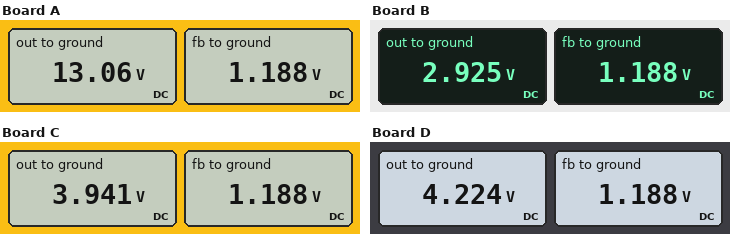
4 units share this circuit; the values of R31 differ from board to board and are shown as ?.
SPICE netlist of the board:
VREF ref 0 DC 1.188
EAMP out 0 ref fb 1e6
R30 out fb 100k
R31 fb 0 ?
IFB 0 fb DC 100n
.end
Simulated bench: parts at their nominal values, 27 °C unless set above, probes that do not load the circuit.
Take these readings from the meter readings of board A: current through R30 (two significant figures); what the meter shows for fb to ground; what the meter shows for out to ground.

120 µA
1.188 V
13.06 V
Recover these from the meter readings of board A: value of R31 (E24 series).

10 kΩ
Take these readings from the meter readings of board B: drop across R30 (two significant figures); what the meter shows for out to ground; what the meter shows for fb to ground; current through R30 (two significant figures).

1.7 V
2.925 V
1.188 V
17 µA
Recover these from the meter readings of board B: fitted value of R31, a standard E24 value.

68 kΩ
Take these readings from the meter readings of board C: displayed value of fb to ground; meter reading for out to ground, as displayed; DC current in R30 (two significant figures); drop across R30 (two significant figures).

1.188 V
3.941 V
28 µA
2.8 V
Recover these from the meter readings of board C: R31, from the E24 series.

43 kΩ
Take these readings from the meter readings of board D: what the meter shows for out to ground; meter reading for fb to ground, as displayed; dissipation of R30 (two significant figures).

4.224 V
1.188 V
92 µW
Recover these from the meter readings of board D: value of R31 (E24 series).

39 kΩ
